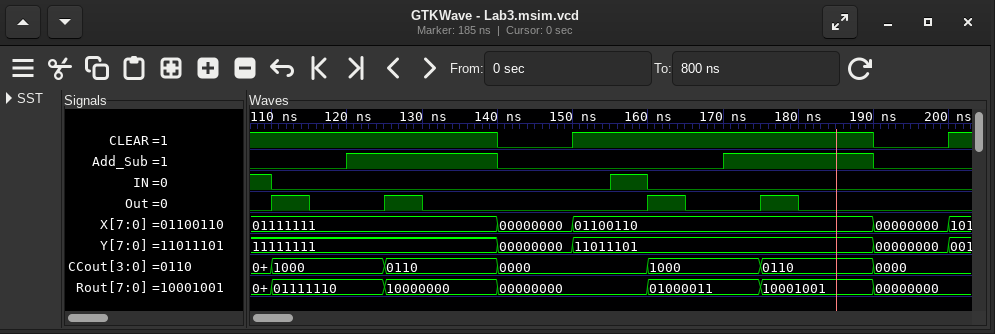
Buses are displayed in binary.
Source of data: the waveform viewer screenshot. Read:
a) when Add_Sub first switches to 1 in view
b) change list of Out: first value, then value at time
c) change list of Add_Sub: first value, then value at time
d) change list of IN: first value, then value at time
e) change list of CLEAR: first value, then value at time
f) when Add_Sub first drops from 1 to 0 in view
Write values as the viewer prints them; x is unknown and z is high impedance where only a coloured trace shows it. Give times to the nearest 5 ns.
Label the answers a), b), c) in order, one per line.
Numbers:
a) 120 ns
b) 0, 1 at 110 ns, 0 at 115 ns, 1 at 125 ns, 0 at 130 ns, 1 at 160 ns, 0 at 165 ns, 1 at 175 ns, 0 at 180 ns
c) 0, 1 at 120 ns, 0 at 140 ns, 1 at 170 ns, 0 at 190 ns
d) 1, 0 at 110 ns, 1 at 155 ns, 0 at 160 ns
e) 1, 0 at 140 ns, 1 at 150 ns, 0 at 190 ns, 1 at 200 ns
f) 140 ns
